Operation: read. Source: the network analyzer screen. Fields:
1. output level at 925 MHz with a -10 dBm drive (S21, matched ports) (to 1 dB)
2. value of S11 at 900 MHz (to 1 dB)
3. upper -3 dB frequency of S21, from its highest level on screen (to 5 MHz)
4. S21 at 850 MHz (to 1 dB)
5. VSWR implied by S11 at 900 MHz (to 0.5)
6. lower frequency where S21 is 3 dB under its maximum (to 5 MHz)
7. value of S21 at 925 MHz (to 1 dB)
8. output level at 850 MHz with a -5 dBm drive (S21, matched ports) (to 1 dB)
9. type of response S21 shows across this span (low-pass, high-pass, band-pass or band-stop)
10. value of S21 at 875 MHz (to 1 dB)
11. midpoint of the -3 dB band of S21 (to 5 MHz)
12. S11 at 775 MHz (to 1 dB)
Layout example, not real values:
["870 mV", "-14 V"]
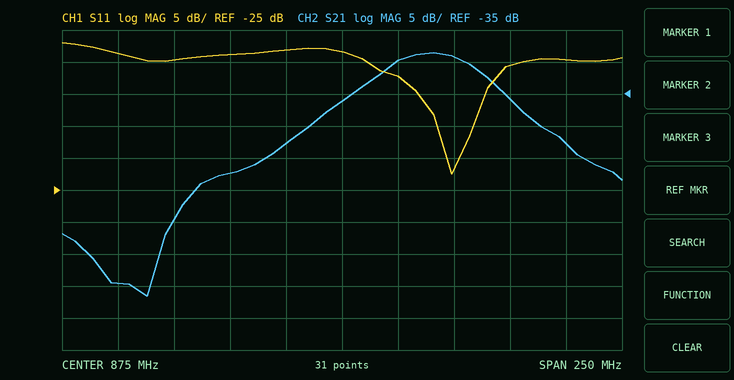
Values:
["-39 dBm", "-7 dB", "935 MHz", "-43 dB", "2.5", "895 MHz", "-29 dB", "-48 dBm", "band-pass", "-36 dB", "915 MHz", "-4 dB"]
